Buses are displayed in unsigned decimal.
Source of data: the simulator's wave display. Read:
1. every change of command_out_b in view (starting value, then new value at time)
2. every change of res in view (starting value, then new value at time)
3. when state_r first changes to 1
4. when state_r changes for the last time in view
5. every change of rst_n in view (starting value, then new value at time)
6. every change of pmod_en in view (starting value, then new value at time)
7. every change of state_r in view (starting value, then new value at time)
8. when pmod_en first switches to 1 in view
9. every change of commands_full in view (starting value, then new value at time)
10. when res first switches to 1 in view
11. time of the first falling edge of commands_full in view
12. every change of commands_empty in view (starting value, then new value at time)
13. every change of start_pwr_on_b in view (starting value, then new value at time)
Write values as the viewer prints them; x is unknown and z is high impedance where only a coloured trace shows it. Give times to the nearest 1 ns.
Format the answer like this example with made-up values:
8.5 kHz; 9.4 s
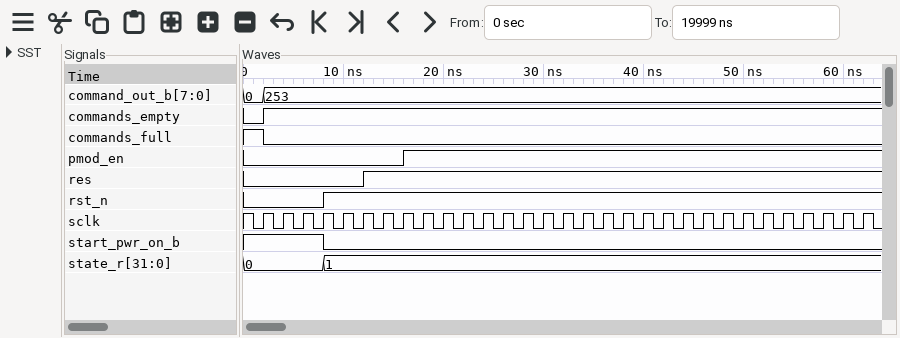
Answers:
0, 253 at 2 ns; 0, 1 at 12 ns; 8 ns; 8 ns; 0, 1 at 8 ns; 0, 1 at 16 ns; 0, 1 at 8 ns; 16 ns; 1, 0 at 2 ns; 12 ns; 2 ns; 0, 1 at 2 ns; 1, 0 at 8 ns
